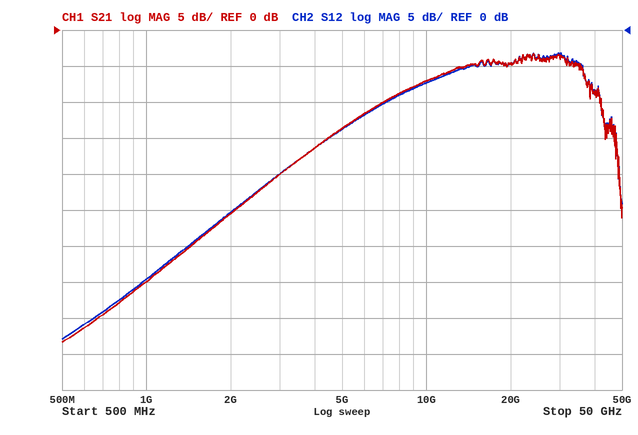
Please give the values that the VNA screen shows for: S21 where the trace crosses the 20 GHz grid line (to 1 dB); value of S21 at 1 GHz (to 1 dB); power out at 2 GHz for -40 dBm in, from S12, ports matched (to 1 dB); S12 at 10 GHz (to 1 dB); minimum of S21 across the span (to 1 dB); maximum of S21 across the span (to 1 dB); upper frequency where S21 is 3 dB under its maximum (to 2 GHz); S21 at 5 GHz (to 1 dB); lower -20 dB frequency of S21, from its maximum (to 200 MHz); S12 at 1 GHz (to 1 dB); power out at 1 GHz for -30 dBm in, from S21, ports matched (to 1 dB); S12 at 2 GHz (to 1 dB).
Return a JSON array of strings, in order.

["-5 dB", "-35 dB", "-65 dBm", "-7 dB", "-43 dB", "-3 dB", "36 GHz", "-14 dB", "2.4 GHz", "-35 dB", "-65 dBm", "-25 dB"]
